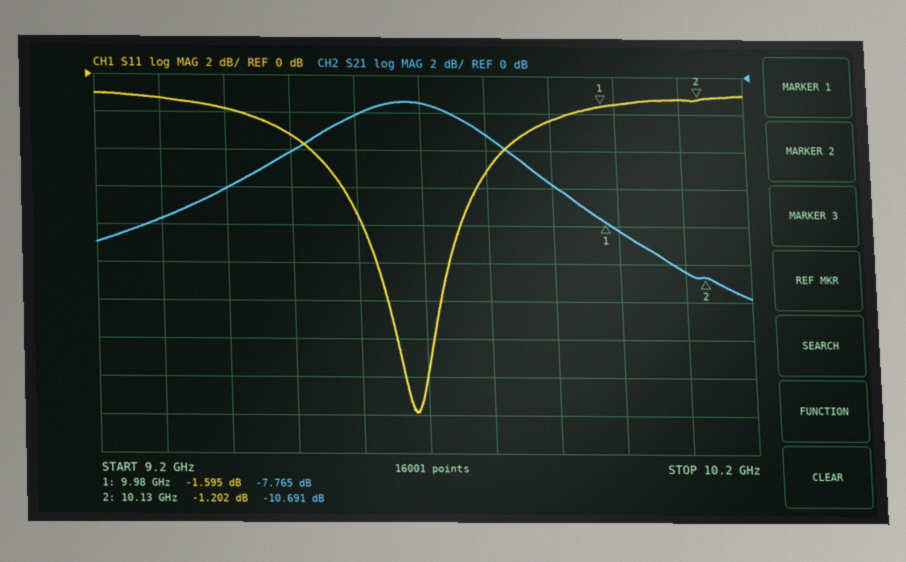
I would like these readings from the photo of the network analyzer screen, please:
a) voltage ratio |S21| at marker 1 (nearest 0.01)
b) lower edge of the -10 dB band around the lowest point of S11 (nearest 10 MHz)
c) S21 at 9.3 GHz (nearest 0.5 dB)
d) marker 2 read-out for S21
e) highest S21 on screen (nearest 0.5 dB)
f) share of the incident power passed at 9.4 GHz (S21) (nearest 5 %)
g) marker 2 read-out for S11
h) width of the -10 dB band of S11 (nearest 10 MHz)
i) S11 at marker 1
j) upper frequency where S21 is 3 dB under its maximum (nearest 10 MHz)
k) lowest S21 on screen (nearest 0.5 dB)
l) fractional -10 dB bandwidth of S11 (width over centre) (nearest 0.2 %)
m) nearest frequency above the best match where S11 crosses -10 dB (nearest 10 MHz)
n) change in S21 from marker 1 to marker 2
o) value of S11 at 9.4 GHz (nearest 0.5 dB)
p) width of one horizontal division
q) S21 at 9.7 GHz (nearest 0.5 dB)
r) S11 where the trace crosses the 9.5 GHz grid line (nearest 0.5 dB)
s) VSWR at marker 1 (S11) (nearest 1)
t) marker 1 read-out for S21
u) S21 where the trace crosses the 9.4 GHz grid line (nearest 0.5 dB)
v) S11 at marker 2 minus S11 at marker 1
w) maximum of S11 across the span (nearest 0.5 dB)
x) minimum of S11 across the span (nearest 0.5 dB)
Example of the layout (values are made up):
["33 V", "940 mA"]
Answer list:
["0.41", "9.63 GHz", "-7.5 dB", "-10.691 dB", "-1.5 dB", "25 %", "-1.202 dB", "110 MHz", "-1.595 dB", "9.85 GHz", "-12.0 dB", "1.2 %", "9.74 GHz", "-2.926 dB", "-2.0 dB", "100 MHz", "-1.5 dB", "-3.0 dB", "11", "-7.765 dB", "-6.0 dB", "0.393 dB", "-1.0 dB", "-18.0 dB"]
